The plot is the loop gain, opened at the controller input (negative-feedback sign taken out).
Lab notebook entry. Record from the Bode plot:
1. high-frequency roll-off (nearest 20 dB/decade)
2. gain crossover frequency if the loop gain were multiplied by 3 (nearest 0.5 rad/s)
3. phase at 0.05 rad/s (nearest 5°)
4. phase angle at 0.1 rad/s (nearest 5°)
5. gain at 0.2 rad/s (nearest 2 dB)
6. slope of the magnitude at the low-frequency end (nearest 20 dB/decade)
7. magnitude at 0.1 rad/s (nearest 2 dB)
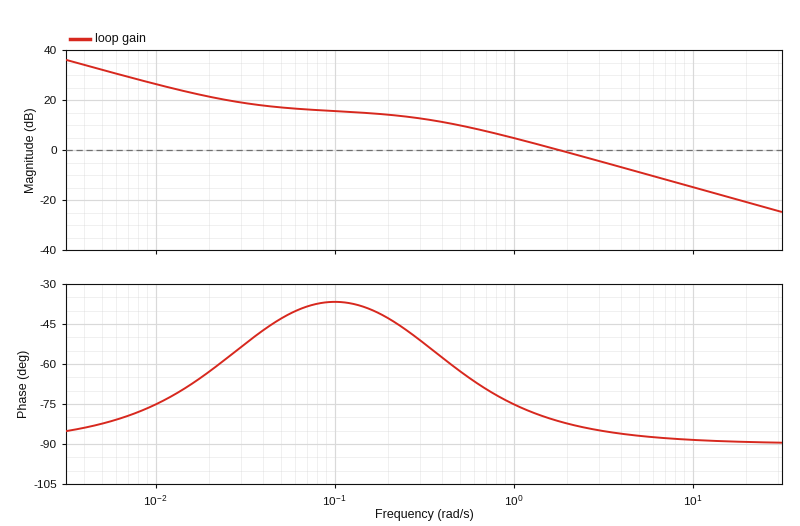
-20 dB/decade
5.5 rad/s
-45°
-35°
14 dB
-20 dB/decade
16 dB
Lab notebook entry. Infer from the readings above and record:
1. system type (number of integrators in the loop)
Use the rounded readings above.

1
